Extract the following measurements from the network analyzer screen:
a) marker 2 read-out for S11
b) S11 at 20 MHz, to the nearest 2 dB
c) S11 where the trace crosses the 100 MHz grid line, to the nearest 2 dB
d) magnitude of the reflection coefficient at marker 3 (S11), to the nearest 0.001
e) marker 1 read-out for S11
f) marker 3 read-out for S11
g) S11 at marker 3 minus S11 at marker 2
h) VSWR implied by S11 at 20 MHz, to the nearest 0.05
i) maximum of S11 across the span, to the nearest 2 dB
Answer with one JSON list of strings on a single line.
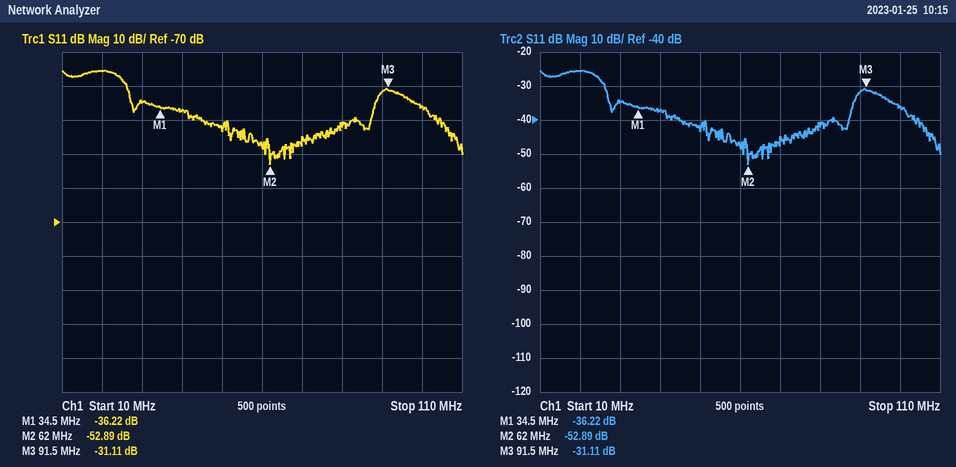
["-52.89 dB", "-26 dB", "-36 dB", "0.028", "-36.22 dB", "-31.11 dB", "21.78 dB", "1.10", "-26 dB"]
